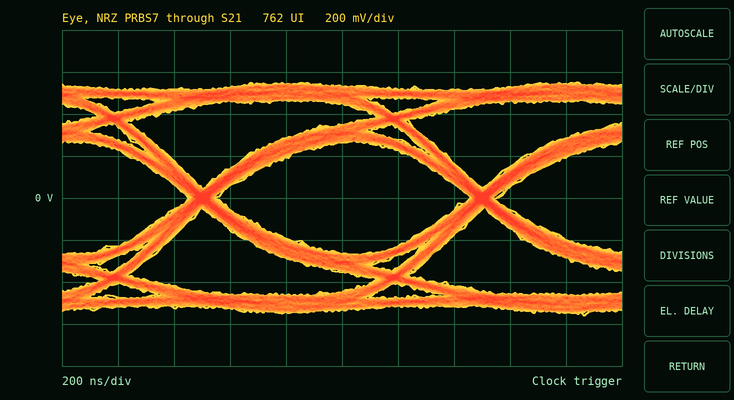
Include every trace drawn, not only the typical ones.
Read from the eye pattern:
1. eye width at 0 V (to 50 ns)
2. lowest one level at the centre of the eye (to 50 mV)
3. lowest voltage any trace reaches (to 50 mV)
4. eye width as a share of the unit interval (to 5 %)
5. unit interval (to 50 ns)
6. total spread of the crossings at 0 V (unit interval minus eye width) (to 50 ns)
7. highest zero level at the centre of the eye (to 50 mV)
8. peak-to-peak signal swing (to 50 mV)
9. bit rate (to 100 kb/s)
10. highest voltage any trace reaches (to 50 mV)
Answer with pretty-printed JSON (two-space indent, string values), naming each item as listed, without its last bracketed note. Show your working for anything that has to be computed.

{
  "eye width at 0 V": "900 ns",
  "lowest one level at the centre of the eye": "250 mV",
  "lowest voltage any trace reaches": "-550 mV",
  "eye width as a share of the unit interval": "900 ns / 1.00 µs ≈ 90 %",
  "unit interval": "1.00 µs",
  "total spread of the crossings at 0 V (unit interval minus eye width)": "100 ns",
  "highest zero level at the centre of the eye": "-250 mV",
  "peak-to-peak signal swing": "1.10 V",
  "bit rate": "1.0 Mb/s",
  "highest voltage any trace reaches": "550 mV"
}
